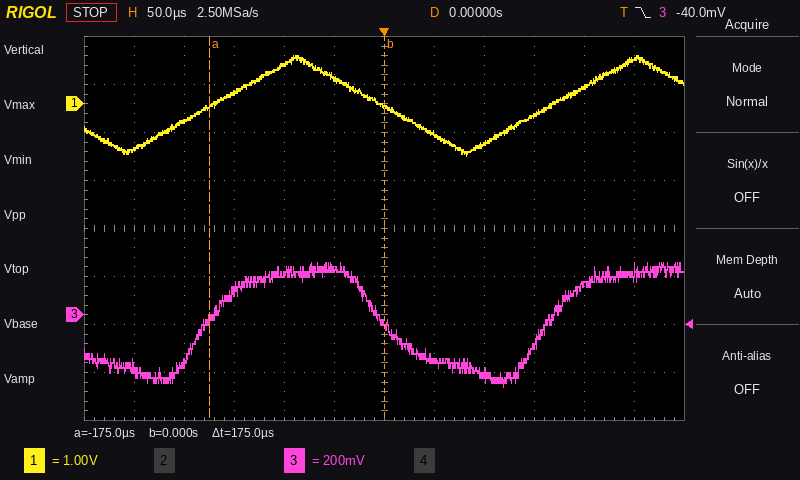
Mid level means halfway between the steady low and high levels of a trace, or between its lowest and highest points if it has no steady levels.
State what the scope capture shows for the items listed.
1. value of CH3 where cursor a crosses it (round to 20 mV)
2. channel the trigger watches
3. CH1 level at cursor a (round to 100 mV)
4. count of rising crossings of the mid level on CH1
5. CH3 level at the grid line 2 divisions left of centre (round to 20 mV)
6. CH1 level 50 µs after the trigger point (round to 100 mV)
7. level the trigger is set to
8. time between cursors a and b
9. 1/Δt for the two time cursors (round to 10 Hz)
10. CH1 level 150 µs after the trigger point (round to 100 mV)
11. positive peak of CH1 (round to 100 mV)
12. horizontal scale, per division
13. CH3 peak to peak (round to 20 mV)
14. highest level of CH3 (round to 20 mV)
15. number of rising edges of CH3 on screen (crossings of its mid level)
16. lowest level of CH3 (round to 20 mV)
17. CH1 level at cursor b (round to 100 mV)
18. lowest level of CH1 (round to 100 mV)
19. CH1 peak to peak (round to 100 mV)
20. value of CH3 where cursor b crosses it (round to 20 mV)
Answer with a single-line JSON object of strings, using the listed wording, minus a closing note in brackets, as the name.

{"value of CH3 where cursor a crosses it": "-20 mV", "channel the trigger watches": "CH3", "CH1 level at cursor a": "-100 mV", "count of rising crossings of the mid level on CH1": "2", "CH3 level at the grid line 2 divisions left of centre": "180 mV", "CH1 level 50 µs after the trigger point": "-600 mV", "level the trigger is set to": "-40.0 mV", "time between cursors a and b": "175 µs", "1/Δt for the two time cursors": "5.71 kHz", "CH1 level 150 µs after the trigger point": "-200 mV", "positive peak of CH1": "1.0 V", "horizontal scale, per division": "50 µs", "CH3 peak to peak": "520 mV", "highest level of CH3": "220 mV", "number of rising edges of CH3 on screen": "2", "lowest level of CH3": "-300 mV", "CH1 level at cursor b": "-100 mV", "lowest level of CH1": "-1.1 V", "CH1 peak to peak": "2.1 V", "value of CH3 where cursor b crosses it": "-40 mV"}
